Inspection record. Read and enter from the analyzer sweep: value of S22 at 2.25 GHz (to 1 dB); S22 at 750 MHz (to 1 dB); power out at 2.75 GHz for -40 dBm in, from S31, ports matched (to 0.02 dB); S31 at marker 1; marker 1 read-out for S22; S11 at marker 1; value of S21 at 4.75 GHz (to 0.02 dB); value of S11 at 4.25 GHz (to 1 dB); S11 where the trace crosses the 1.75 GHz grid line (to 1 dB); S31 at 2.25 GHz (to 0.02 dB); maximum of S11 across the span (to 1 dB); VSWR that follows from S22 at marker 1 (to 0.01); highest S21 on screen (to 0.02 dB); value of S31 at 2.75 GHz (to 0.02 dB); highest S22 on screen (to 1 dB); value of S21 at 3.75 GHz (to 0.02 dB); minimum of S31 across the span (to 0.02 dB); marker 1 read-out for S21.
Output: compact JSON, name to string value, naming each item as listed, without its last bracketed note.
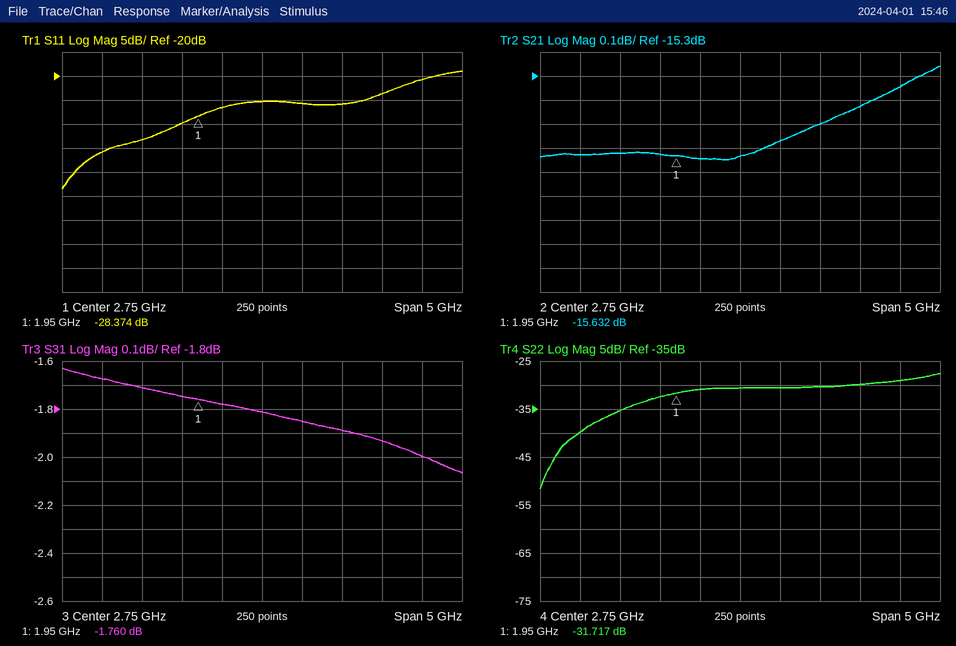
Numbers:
{"value of S22 at 2.25 GHz": "-31 dB", "S22 at 750 MHz": "-40 dB", "power out at 2.75 GHz for -40 dBm in, from S31, ports matched": "-41.82 dBm", "S31 at marker 1": "-1.760 dB", "marker 1 read-out for S22": "-31.717 dB", "S11 at marker 1": "-28.374 dB", "value of S21 at 4.75 GHz": "-15.34 dB", "value of S11 at 4.25 GHz": "-24 dB", "S11 where the trace crosses the 1.75 GHz grid line": "-30 dB", "S31 at 2.25 GHz": "-1.78 dB", "maximum of S11 across the span": "-19 dB", "VSWR that follows from S22 at marker 1": "1.05", "highest S21 on screen": "-15.26 dB", "value of S31 at 2.75 GHz": "-1.82 dB", "highest S22 on screen": "-28 dB", "value of S21 at 3.75 GHz": "-15.50 dB", "minimum of S31 across the span": "-2.06 dB", "marker 1 read-out for S21": "-15.632 dB"}
